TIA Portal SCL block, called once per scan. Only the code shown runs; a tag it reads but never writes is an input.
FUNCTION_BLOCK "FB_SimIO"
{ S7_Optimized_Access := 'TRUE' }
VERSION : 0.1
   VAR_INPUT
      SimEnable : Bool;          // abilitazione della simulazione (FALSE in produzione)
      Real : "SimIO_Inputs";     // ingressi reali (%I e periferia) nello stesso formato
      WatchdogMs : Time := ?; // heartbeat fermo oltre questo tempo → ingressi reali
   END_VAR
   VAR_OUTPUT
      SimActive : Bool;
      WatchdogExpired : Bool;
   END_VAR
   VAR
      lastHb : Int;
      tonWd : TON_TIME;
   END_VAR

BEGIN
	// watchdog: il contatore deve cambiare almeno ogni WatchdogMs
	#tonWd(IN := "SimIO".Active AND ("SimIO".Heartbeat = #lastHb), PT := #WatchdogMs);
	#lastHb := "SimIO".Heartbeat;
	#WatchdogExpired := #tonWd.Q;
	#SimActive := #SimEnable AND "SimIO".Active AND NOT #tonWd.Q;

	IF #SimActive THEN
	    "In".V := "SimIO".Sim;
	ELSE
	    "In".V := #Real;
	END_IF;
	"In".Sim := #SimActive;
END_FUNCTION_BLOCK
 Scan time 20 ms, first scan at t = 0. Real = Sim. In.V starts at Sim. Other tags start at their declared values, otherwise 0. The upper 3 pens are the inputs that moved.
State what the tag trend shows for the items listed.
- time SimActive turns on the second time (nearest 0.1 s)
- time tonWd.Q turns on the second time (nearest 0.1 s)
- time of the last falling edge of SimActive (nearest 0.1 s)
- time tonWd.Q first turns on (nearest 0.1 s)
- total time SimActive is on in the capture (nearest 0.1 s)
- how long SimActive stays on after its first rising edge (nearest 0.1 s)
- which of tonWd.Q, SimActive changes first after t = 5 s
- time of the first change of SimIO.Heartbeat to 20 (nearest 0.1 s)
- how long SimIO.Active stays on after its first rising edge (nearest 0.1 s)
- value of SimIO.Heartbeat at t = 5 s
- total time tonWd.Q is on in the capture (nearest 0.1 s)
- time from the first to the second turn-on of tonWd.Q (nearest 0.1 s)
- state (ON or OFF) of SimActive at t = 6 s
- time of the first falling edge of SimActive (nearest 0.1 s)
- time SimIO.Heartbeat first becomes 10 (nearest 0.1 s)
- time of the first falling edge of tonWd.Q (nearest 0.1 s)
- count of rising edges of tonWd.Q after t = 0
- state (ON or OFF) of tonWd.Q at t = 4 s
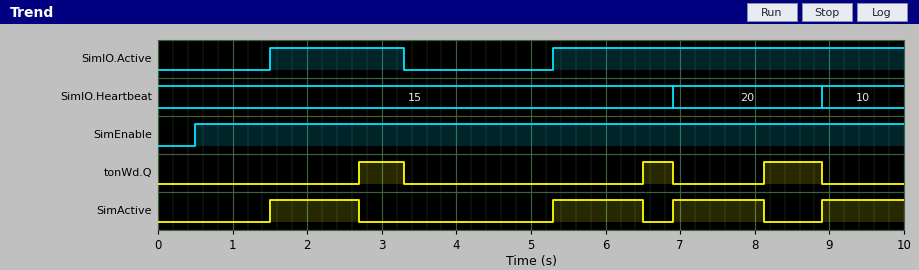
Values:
5.3 s
6.5 s
8.1 s
2.7 s
4.7 s
1.2 s
SimActive
6.9 s
1.8 s
15
1.8 s
3.8 s
ON
2.7 s
8.9 s
3.3 s
3
OFF
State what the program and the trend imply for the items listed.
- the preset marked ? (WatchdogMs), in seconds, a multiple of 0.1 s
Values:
1.2 s
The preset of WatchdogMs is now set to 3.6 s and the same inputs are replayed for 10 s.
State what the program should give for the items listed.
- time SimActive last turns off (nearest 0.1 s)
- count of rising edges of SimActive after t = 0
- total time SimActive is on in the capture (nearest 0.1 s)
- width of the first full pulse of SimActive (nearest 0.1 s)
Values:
3.3 s
2
6.5 s
1.8 s
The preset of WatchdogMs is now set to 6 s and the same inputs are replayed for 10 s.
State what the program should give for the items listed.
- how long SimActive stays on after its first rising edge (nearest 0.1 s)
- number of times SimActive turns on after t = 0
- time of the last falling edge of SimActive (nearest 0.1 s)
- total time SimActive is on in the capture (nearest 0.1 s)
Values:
1.8 s
2
3.3 s
6.5 s
